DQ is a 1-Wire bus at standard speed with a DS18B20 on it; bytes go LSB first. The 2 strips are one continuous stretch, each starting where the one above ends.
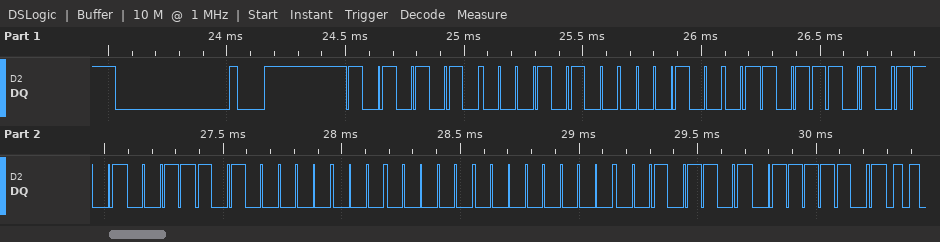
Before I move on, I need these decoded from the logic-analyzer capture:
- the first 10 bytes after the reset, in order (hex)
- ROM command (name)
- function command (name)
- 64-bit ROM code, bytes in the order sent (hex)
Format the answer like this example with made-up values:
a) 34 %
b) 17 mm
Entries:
a) 55 28 88 5D CB 05 00 00 B4 BE
b) Match ROM
c) Read Scratchpad
d) 28 88 5D CB 05 00 00 B4
